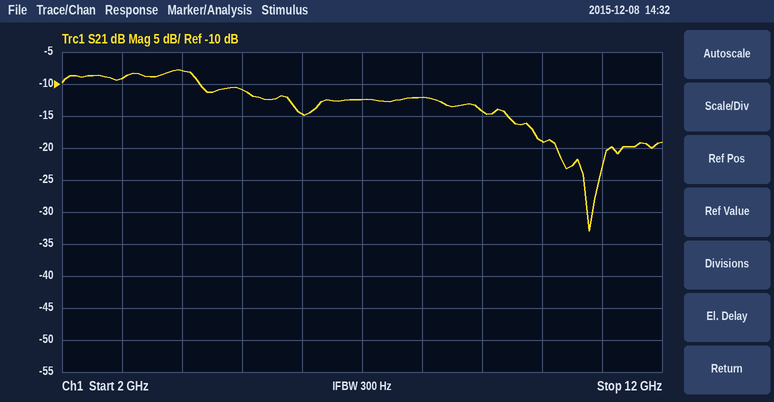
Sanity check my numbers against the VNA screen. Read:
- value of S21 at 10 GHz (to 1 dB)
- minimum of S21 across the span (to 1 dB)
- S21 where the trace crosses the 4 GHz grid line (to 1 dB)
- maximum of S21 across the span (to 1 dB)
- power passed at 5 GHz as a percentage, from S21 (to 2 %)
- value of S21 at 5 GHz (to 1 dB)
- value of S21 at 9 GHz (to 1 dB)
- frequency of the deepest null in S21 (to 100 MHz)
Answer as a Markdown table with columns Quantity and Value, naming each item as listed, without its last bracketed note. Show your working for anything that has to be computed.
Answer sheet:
| Quantity | Value |
|---|---|
| value of S21 at 10 GHz | -19 dB |
| minimum of S21 across the span | -33 dB |
| S21 where the trace crosses the 4 GHz grid line | -8 dB |
| maximum of S21 across the span | -8 dB |
| power passed at 5 GHz as a percentage, from S21 | 10^(-11/10) ≈ 8 % |
| value of S21 at 5 GHz | -11 dB |
| value of S21 at 9 GHz | -14 dB |
| frequency of the deepest null in S21 | 10.8 GHz |
